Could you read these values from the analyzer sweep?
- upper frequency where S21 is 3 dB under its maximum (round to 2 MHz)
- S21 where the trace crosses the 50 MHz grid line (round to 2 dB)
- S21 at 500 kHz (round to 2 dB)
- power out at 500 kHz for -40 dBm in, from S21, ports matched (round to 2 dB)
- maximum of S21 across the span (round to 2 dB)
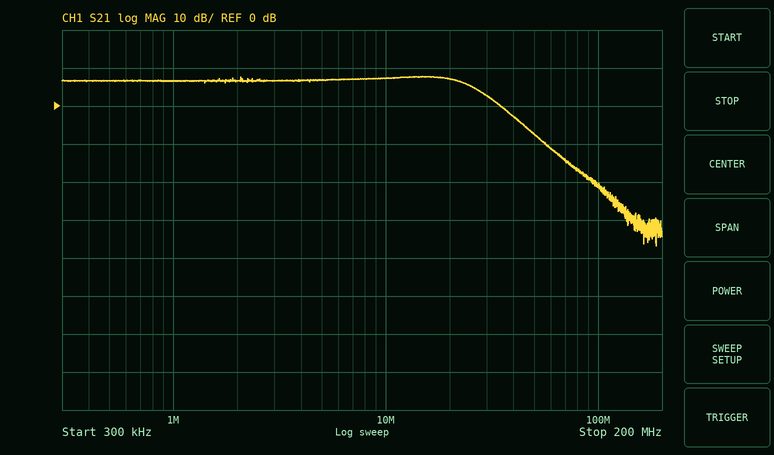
26 MHz
-8 dB
6 dB
-34 dBm
8 dB
